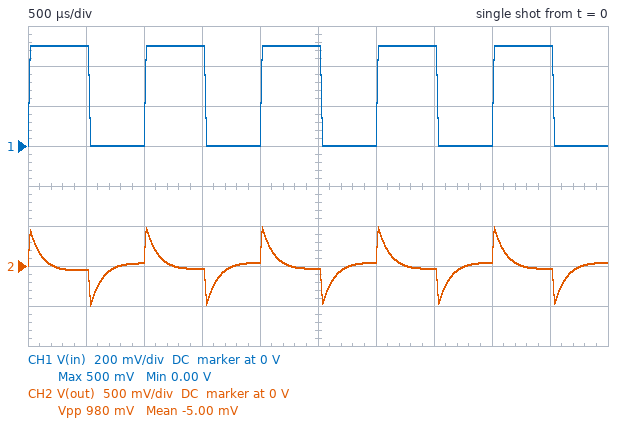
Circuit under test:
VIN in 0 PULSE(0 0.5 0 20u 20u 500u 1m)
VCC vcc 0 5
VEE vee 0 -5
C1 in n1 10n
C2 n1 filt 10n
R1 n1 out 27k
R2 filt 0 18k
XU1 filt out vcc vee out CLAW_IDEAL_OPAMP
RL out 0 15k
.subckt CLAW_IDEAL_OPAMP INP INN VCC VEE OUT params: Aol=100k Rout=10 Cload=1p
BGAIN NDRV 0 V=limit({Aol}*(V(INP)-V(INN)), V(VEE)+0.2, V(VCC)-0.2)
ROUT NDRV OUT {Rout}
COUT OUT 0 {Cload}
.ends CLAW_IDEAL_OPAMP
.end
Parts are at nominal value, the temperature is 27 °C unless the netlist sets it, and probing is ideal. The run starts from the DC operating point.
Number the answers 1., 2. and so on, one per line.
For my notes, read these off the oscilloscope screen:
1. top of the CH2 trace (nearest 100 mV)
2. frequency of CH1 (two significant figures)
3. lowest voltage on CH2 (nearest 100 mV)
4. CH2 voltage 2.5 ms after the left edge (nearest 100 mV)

1. 500 mV
2. 1.0 kHz
3. -500 mV
4. 0 V
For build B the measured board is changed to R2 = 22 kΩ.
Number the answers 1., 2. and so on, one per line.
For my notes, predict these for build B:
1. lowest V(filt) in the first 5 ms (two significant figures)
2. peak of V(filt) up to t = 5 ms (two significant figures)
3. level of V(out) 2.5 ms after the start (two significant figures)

1. -510 mV
2. 500 mV
3. -39 mV
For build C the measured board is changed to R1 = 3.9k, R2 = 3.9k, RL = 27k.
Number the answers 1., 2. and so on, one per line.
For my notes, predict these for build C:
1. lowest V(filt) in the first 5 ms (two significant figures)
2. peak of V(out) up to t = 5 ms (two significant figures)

1. -300 mV
2. 300 mV
